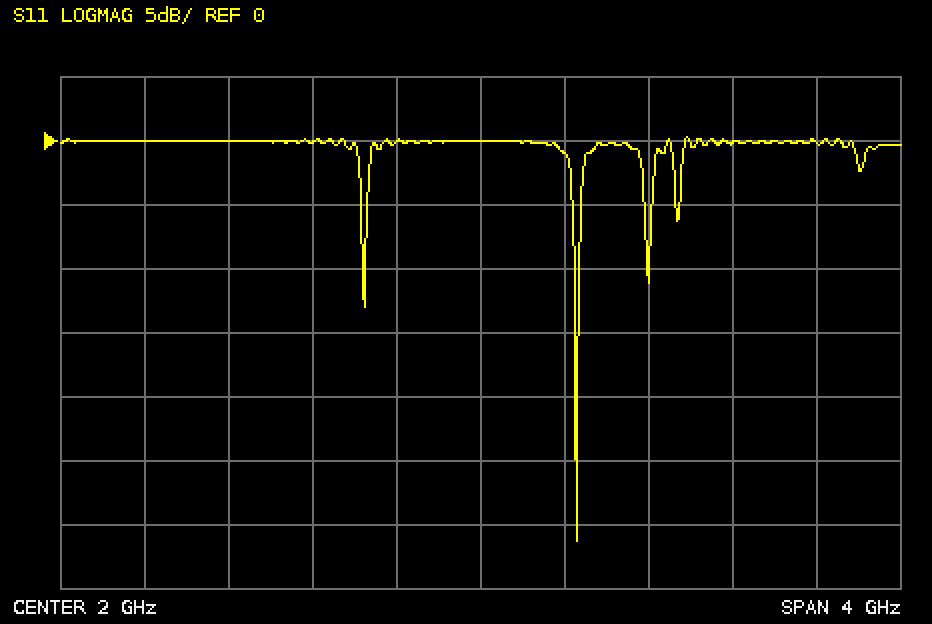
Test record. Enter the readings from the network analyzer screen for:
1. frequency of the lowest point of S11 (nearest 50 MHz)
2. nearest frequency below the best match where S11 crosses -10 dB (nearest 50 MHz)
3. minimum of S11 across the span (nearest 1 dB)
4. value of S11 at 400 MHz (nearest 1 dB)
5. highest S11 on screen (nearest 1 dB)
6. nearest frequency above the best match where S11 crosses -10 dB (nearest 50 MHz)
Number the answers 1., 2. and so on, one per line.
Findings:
1. 2.45 GHz
2. 2.45 GHz
3. -31 dB
4. 0 dB
5. 0 dB
6. 2.45 GHz
